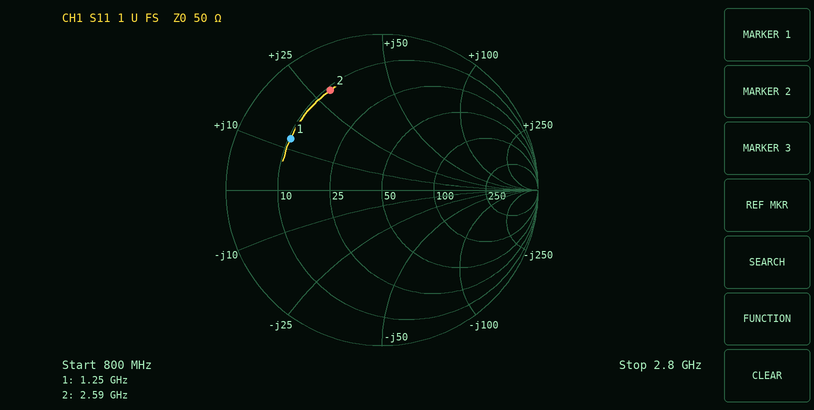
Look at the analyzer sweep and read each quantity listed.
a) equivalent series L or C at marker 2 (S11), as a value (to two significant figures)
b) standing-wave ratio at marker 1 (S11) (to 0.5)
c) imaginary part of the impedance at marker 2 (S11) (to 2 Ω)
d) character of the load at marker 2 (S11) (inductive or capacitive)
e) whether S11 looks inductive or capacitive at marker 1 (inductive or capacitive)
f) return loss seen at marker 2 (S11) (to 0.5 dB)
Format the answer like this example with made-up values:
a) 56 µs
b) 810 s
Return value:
a) 1.8 nH
b) 5.0
c) +30 Ω
d) inductive
e) inductive
f) 3.0 dB
